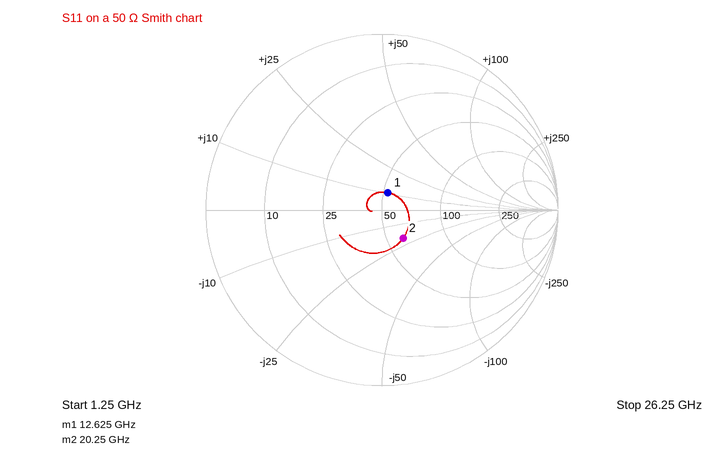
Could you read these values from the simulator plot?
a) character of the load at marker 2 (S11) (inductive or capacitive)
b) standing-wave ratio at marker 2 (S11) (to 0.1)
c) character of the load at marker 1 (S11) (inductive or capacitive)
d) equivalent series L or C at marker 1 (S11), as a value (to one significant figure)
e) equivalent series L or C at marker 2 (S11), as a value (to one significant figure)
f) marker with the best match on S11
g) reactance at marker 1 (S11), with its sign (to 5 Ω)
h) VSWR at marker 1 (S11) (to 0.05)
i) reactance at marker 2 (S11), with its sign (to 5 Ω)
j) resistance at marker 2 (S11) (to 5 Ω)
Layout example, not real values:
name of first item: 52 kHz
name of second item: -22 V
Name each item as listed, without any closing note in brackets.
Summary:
character of the load at marker 2 (S11): capacitive
standing-wave ratio at marker 2 (S11): 1.5
character of the load at marker 1 (S11): inductive
equivalent series L or C at marker 1 (S11), as a value: 100 pH
equivalent series L or C at marker 2 (S11), as a value: 400 fF
marker with the best match on S11: marker 1
reactance at marker 1 (S11), with its sign: +10 Ω
VSWR at marker 1 (S11): 1.25
reactance at marker 2 (S11), with its sign: -20 Ω
resistance at marker 2 (S11): 60 Ω
